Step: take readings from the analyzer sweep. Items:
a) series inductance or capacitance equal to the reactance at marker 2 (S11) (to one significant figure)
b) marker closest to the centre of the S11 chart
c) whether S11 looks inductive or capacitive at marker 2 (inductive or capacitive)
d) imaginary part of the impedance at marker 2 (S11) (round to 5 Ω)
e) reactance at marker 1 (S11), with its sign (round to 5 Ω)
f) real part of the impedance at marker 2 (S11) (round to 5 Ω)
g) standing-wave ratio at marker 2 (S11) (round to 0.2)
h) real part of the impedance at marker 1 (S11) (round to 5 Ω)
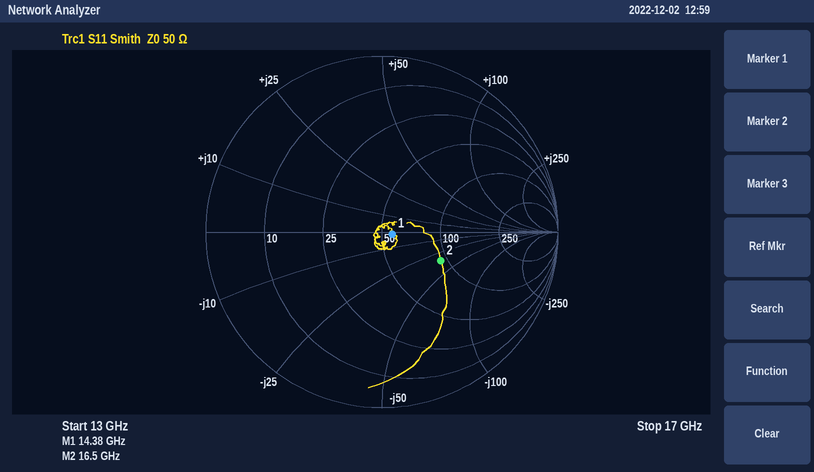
300 fF
marker 1
capacitive
-35 Ω
0 Ω
90 Ω
2.2
55 Ω
